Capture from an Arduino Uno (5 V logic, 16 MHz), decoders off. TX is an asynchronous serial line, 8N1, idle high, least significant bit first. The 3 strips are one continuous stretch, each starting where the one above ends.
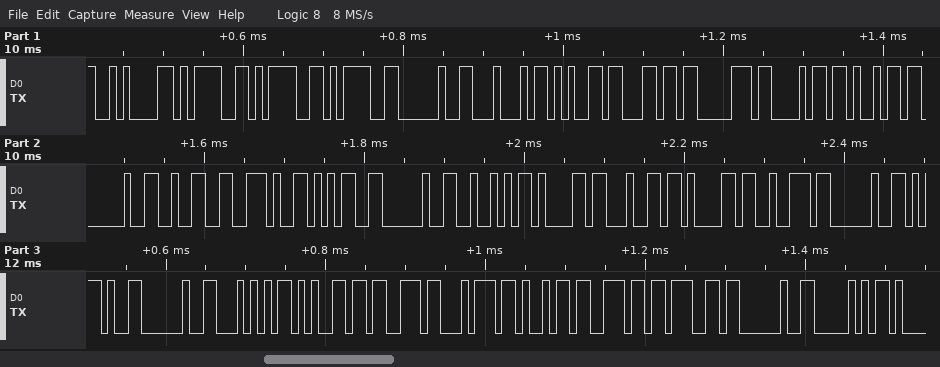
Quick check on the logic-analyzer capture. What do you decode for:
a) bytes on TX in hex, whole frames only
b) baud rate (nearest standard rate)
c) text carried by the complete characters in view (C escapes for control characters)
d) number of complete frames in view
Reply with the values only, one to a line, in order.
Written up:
0A 3D 3D 3D 20 44 65 6C 70 68 69 20 32 2E 35 20 52 61 64 61 72 20 2D 20 54 65 73 74 69 6E 67 20 50
115200 baud
"\n=== Delphi 2.5 Radar - Testing P"
33
